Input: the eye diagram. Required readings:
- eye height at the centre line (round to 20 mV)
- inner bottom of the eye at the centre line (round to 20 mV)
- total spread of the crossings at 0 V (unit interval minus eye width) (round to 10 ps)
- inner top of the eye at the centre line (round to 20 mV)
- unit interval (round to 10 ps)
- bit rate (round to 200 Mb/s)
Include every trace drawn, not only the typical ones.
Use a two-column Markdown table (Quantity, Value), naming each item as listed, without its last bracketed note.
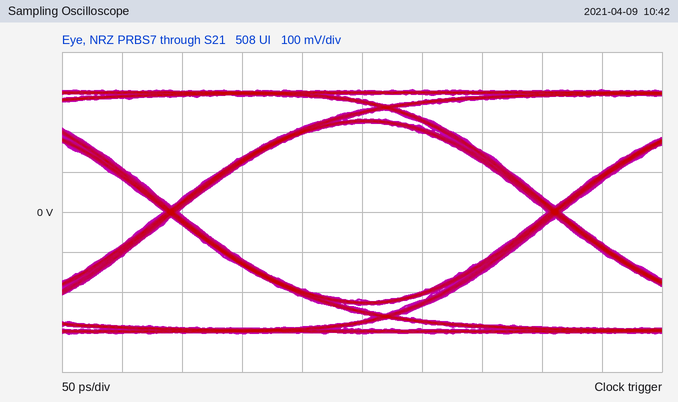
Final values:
| Quantity | Value |
|---|---|
| eye height at the centre line | 440 mV |
| inner bottom of the eye at the centre line | -220 mV |
| total spread of the crossings at 0 V (unit interval minus eye width) | 10 ps |
| inner top of the eye at the centre line | 220 mV |
| unit interval | 320 ps |
| bit rate | 3.2 Gb/s |
